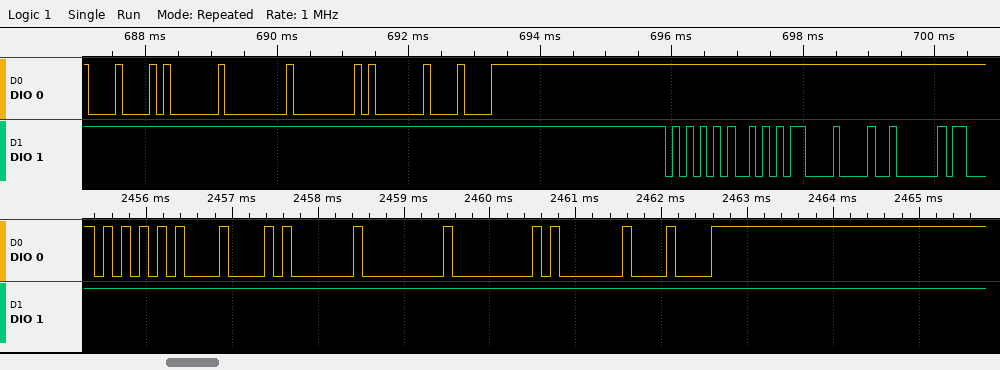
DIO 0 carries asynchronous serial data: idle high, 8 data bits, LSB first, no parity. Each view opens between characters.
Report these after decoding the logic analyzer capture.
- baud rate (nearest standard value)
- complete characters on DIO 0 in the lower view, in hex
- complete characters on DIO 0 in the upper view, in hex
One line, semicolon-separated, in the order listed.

9600 baud; 55, 08, 01, 00, 00, 01, 08; 08, 01, 00, 00, 01, 08
